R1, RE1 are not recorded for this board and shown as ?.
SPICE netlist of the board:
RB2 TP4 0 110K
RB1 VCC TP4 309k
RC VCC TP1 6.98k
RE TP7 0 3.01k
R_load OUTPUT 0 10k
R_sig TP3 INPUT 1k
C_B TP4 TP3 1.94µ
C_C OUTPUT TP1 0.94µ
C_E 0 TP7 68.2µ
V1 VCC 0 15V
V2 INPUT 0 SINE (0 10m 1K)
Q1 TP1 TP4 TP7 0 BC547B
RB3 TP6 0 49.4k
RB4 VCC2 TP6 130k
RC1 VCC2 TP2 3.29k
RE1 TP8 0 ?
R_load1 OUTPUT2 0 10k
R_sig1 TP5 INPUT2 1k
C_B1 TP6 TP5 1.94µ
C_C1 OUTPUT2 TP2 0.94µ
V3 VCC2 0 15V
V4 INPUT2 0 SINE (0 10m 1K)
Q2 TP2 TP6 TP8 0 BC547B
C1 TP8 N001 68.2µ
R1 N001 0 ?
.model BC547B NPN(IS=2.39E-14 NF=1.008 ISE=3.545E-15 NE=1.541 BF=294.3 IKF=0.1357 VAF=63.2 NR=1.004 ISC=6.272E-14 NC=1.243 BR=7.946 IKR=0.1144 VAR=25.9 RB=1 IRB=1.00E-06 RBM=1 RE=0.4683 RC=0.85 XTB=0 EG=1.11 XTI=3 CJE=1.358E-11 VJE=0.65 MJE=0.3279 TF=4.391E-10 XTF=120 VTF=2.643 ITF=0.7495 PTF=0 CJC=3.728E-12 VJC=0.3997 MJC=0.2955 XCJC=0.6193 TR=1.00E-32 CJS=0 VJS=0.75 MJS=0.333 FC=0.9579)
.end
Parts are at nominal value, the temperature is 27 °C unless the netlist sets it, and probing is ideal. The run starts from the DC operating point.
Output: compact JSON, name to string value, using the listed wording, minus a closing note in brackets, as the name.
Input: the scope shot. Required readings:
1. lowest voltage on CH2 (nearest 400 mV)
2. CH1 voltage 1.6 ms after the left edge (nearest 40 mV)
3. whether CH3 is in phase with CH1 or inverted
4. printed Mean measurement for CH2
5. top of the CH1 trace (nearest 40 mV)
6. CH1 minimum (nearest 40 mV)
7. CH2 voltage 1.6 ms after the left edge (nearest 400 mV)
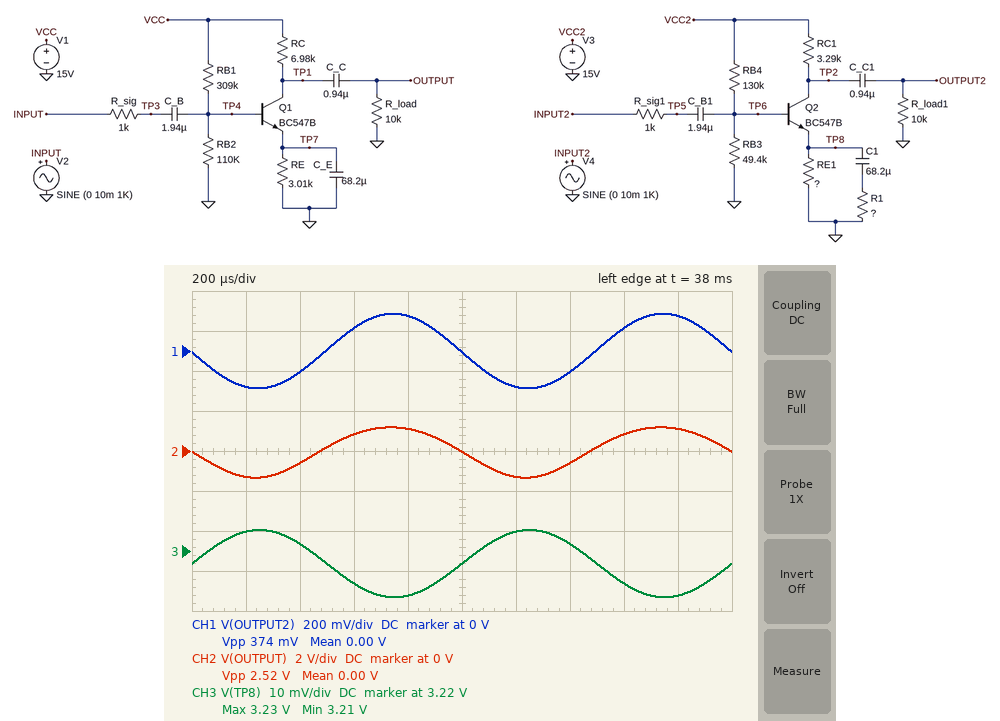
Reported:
{"lowest voltage on CH2": "-1.2 V", "CH1 voltage 1.6 ms after the left edge": "120 mV", "whether CH3 is in phase with CH1 or inverted": "inverted", "printed Mean measurement for CH2": "0.00 V", "top of the CH1 trace": "200 mV", "CH1 minimum": "-200 mV", "CH2 voltage 1.6 ms after the left edge": "800 mV"}
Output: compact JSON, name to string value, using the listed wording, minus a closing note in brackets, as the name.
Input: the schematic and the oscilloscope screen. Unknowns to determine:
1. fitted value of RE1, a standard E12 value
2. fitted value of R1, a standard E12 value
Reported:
{"fitted value of RE1, a standard E12 value": "1.5 kΩ", "fitted value of R1, a standard E12 value": "120 Ω"}
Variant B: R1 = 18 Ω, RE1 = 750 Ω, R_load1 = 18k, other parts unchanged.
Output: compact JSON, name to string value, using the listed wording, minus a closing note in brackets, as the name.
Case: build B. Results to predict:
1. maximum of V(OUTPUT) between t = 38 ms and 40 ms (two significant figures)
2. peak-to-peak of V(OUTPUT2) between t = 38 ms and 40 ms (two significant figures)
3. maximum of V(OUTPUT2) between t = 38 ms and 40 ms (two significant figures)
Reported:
{"maximum of V(OUTPUT) between t = 38 ms and 40 ms": "1.2 V", "peak-to-peak of V(OUTPUT2) between t = 38 ms and 40 ms": "380 mV", "maximum of V(OUTPUT2) between t = 38 ms and 40 ms": "290 mV"}
